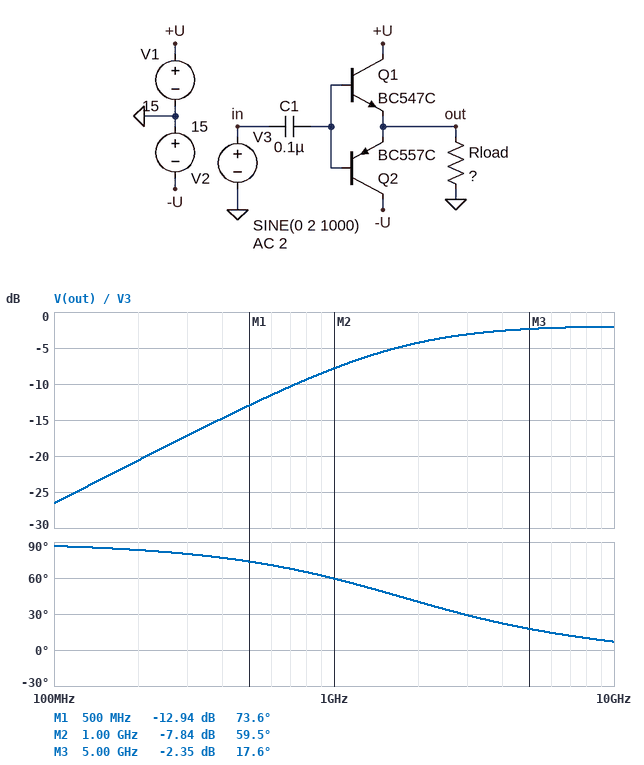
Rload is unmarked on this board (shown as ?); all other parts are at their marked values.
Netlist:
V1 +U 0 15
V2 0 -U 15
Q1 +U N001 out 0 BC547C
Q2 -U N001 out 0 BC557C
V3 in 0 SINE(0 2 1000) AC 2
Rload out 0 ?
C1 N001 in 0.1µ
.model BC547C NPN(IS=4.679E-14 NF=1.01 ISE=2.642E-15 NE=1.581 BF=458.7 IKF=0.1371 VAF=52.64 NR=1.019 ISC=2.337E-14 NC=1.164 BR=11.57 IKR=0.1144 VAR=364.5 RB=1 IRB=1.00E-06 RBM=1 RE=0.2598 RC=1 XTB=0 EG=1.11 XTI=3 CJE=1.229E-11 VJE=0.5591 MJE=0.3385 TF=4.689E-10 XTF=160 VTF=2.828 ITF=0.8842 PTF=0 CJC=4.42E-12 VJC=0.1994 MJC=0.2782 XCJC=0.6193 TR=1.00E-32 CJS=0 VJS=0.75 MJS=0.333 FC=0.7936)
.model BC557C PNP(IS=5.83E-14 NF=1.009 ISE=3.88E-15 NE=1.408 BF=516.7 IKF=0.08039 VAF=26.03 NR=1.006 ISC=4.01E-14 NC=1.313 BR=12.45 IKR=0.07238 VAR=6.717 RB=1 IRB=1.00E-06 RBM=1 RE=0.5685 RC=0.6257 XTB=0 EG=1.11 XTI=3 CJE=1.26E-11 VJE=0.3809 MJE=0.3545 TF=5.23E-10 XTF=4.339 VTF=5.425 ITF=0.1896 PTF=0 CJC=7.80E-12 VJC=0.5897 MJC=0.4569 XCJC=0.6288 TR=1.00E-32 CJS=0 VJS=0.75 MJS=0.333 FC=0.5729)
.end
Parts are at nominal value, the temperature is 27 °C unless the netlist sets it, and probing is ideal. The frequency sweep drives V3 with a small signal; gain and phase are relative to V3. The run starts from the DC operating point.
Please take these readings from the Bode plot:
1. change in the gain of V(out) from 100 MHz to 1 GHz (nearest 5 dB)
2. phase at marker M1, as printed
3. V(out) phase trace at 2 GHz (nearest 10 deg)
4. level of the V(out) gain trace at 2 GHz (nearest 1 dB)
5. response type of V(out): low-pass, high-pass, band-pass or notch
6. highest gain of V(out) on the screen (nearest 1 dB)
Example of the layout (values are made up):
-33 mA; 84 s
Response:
20 dB; 73.6 deg; 40 deg; -4 dB; high-pass; -2 dB
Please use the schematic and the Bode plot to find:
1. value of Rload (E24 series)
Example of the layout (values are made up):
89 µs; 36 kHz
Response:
3 Ω
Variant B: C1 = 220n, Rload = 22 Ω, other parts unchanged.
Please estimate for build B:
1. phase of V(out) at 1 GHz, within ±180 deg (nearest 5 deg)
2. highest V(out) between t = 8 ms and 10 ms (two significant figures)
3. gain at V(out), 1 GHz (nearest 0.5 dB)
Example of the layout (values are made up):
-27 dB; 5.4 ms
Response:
15 deg; 1.2 V; -0.5 dB
